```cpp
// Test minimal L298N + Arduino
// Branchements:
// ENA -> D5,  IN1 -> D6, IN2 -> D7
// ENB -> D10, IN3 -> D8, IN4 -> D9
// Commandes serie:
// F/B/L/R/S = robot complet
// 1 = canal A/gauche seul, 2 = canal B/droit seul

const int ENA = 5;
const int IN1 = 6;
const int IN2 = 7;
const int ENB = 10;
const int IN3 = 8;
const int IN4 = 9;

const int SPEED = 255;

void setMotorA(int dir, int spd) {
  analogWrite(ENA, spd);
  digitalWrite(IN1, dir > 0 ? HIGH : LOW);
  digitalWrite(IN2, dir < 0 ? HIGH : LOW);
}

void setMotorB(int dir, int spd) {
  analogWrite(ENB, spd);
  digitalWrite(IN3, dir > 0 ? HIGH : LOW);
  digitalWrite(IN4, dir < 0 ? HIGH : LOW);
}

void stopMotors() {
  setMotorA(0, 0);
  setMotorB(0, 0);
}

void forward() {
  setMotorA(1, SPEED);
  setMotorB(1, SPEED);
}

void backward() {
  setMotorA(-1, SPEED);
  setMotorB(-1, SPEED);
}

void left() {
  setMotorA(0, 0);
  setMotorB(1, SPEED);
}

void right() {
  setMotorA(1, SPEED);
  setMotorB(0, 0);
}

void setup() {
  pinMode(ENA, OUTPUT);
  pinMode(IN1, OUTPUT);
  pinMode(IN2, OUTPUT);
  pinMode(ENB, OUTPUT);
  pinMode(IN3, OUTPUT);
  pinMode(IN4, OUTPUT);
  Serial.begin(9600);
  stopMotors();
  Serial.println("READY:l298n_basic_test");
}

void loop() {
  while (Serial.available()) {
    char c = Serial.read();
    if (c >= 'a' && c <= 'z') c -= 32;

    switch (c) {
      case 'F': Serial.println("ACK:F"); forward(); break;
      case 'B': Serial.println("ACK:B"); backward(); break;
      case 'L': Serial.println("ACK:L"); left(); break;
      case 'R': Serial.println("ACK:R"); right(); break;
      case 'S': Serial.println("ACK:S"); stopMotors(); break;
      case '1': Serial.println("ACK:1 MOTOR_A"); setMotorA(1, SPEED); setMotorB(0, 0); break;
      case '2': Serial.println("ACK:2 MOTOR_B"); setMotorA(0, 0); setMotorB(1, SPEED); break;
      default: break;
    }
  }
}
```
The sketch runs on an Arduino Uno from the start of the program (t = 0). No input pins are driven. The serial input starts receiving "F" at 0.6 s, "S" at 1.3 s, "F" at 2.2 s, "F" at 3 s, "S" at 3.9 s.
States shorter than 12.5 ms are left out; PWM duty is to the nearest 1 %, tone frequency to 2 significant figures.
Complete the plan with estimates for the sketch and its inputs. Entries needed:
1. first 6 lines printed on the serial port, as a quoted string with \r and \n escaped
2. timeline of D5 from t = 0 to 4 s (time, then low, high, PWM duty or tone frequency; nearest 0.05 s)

"READY:l298n_basic_test\r\nACK:F\r\nACK:S\r\nACK:F\r\nACK:F\r\nACK:S\r\n"
0 s low; 0.6 s high; 1.3 s low; 2.2 s high; 3.9 s low
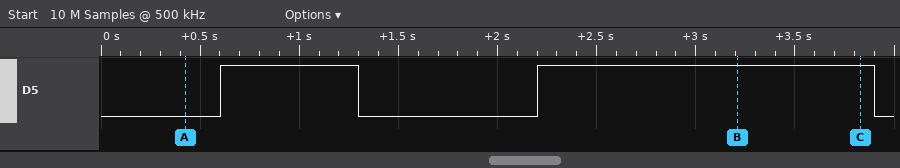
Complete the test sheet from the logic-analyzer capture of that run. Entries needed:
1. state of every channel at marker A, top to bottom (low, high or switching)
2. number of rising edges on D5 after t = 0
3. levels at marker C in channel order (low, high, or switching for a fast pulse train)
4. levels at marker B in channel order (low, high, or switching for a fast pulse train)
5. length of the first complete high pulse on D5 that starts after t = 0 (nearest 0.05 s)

D5 low
2
D5 high
D5 high
0.70 s
